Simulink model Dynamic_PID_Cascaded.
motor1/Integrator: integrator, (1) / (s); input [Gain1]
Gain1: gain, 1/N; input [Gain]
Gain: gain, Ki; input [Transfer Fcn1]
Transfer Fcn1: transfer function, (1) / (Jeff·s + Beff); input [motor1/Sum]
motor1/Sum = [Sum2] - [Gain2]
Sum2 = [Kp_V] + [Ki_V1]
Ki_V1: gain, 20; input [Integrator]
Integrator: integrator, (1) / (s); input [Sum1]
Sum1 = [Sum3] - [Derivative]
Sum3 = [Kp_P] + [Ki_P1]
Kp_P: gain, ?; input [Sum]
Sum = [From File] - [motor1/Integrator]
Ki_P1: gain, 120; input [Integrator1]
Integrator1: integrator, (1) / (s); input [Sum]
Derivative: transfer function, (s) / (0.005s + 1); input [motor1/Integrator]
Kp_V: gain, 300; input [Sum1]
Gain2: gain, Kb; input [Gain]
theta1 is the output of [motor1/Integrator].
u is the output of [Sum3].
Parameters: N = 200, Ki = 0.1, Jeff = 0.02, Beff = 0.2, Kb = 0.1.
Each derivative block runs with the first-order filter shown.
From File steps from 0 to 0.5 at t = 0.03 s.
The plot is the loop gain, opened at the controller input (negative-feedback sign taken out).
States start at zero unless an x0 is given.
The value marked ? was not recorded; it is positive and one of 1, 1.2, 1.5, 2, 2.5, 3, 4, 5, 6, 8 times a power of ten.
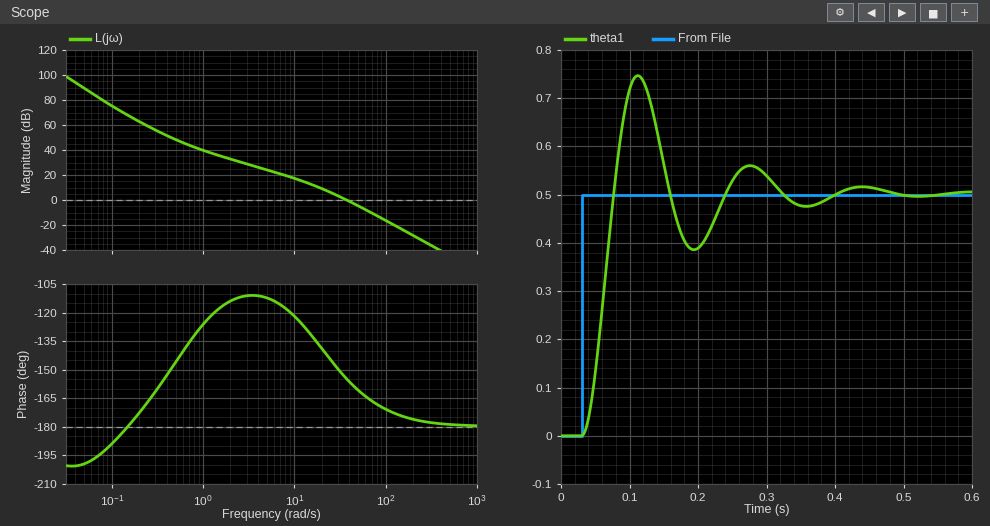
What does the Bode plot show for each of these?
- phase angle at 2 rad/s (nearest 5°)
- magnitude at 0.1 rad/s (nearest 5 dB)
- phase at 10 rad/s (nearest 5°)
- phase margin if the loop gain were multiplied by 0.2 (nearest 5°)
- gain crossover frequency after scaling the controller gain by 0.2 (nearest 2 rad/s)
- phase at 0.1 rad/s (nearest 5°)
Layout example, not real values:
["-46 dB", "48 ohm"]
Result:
["-115°", "75 dB", "-120°", "50°", "14 rad/s", "-190°"]
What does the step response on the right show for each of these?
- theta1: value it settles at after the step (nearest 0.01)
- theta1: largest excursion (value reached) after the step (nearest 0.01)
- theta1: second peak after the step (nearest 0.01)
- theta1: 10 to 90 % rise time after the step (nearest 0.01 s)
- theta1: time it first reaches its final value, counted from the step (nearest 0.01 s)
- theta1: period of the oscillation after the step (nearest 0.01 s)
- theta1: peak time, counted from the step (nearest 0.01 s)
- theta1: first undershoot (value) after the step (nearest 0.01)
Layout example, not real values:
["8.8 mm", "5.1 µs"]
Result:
["0.50", "0.75", "0.56", "0.03 s", "0.05 s", "0.16 s", "0.08 s", "0.39"]
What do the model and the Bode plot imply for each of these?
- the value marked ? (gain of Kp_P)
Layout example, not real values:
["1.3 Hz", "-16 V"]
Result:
["200"]
